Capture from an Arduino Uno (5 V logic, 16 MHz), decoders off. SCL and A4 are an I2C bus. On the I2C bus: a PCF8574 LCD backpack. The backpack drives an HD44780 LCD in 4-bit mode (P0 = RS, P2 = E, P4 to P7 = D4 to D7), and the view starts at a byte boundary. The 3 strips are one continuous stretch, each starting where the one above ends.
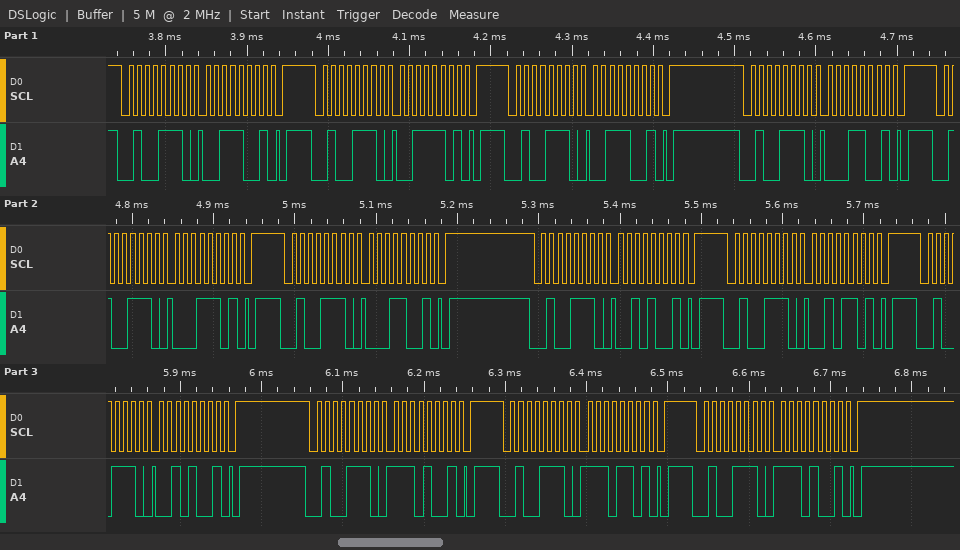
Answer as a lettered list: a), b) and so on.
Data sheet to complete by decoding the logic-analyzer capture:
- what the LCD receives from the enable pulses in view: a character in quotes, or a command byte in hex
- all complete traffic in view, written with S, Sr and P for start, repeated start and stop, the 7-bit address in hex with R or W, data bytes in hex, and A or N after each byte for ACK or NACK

a) '1' '.'
b) S 27W A 39 A P S 27W A 3D A P S 27W A 39 A P S 27W A 19 A P S 27W A 1D A P S 27W A 19 A P S 27W A 29 A P S 27W A 2D A P S 27W A 29 A P S 27W A E9 A P S 27W A ED A P S 27W A E9 A P
